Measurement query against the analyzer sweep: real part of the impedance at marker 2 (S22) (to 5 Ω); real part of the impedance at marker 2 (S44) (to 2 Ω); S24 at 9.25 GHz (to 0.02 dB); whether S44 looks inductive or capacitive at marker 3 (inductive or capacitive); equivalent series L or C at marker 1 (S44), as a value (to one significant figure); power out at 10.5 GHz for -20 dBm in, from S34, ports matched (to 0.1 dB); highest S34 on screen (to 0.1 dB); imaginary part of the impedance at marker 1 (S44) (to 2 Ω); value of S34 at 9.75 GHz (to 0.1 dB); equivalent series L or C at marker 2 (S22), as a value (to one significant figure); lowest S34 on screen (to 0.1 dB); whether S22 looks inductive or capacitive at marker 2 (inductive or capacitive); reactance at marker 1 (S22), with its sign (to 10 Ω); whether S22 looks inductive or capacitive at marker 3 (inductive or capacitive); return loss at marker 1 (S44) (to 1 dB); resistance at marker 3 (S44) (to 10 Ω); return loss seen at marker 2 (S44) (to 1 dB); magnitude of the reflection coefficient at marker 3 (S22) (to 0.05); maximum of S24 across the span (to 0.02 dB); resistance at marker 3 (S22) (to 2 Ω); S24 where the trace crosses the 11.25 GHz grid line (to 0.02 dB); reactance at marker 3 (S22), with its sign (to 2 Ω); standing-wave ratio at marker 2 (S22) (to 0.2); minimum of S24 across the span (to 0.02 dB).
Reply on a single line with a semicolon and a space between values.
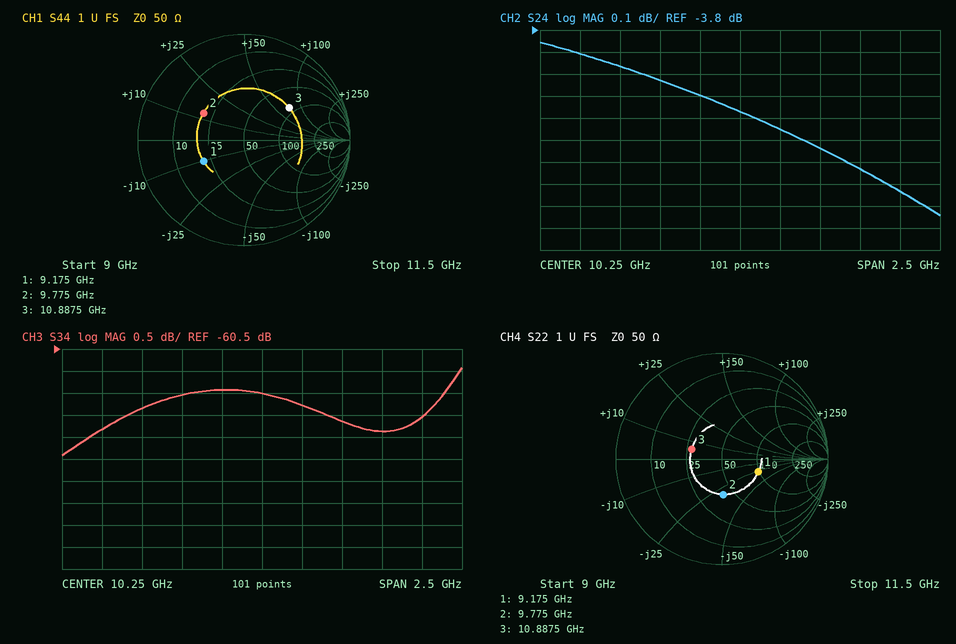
40 Ω; 20 Ω; -3.90 dB; inductive; 2 pF; -81.8 dBm; -60.9 dB; -10 Ω; -61.5 dB; 500 fF; -62.9 dB; capacitive; -30 Ω; inductive; 7 dB; 90 Ω; 7 dB; 0.30; -3.86 dB; 28 Ω; -4.54 dB; +6 Ω; 2.0; -4.64 dB
